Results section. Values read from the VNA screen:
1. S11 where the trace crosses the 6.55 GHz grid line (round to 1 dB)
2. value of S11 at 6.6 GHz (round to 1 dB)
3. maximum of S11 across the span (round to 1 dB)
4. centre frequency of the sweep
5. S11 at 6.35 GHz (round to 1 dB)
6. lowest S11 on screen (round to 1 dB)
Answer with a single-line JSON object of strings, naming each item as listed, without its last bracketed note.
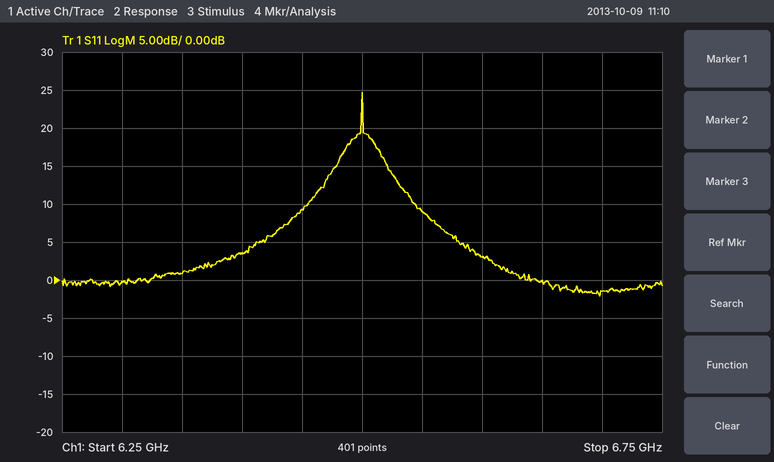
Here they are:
{"S11 where the trace crosses the 6.55 GHz grid line": "9 dB", "value of S11 at 6.6 GHz": "3 dB", "maximum of S11 across the span": "25 dB", "centre frequency of the sweep": "6.5 GHz", "S11 at 6.35 GHz": "1 dB", "lowest S11 on screen": "-2 dB"}
